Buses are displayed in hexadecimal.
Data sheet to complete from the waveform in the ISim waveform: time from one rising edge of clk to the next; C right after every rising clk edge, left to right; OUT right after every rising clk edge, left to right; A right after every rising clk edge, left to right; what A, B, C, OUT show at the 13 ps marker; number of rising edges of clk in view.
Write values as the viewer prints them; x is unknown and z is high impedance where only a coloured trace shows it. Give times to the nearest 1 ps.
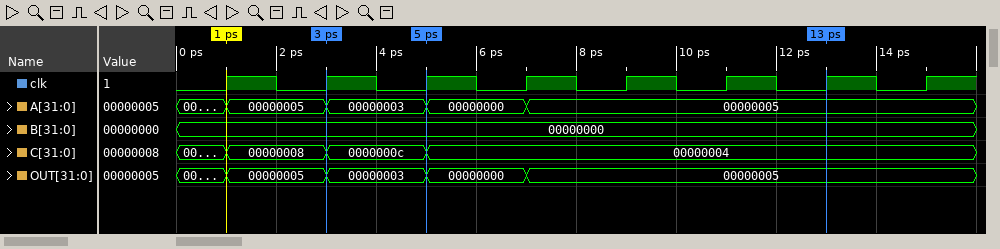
2 ps
00000008, 0000000c, 00000004, 00000004, 00000004, 00000004, 00000004, 00000004
00000005, 00000003, 00000000, 00000005, 00000005, 00000005, 00000005, 00000005
00000005, 00000003, 00000000, 00000005, 00000005, 00000005, 00000005, 00000005
A=00000005, B=00000000, C=00000004, OUT=00000005
8
